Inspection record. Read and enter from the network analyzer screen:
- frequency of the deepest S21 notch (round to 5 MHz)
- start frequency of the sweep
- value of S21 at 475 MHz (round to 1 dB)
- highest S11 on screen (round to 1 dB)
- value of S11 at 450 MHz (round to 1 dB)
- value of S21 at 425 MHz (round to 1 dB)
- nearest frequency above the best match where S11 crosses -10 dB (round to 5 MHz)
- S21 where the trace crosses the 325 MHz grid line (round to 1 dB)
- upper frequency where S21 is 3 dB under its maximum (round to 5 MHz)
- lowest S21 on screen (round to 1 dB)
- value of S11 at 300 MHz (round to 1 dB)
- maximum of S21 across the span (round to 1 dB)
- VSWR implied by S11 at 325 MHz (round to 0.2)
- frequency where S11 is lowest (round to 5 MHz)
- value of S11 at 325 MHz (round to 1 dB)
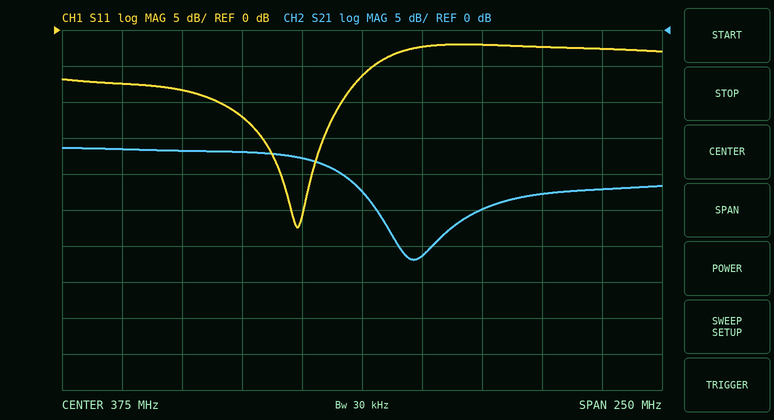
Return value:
395 MHz
250 MHz
-22 dB
-2 dB
-2 dB
-25 dB
365 MHz
-17 dB
365 MHz
-32 dB
-8 dB
-16 dB
1.6
350 MHz
-12 dB
